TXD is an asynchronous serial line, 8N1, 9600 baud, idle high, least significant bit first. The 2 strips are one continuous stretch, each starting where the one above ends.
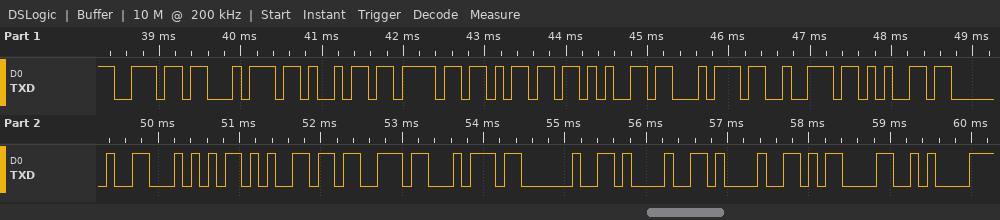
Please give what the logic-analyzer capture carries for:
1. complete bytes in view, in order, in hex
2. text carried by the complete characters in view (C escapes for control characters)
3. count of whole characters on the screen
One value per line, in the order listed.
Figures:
6E 74 69 6F 6D 65 74 72 65 20 54 65 73 74 20 21 21 0D 0A
"ntiometre Test !!\r\n"
19
